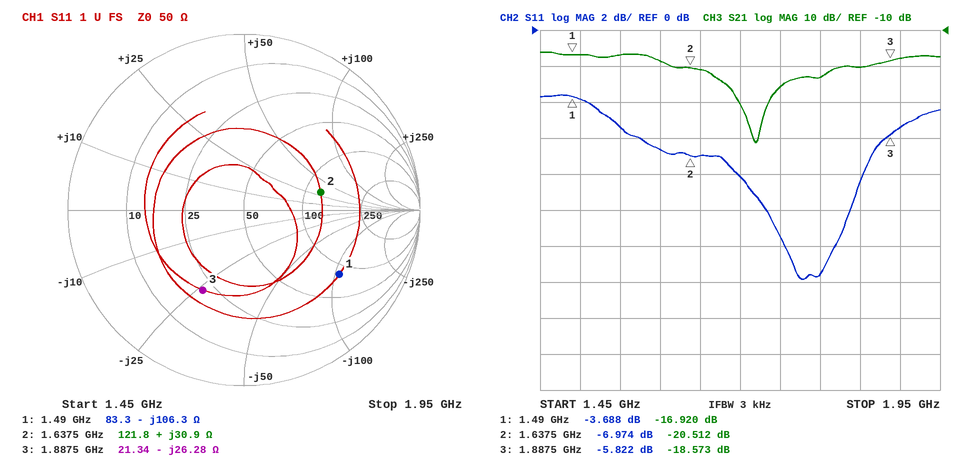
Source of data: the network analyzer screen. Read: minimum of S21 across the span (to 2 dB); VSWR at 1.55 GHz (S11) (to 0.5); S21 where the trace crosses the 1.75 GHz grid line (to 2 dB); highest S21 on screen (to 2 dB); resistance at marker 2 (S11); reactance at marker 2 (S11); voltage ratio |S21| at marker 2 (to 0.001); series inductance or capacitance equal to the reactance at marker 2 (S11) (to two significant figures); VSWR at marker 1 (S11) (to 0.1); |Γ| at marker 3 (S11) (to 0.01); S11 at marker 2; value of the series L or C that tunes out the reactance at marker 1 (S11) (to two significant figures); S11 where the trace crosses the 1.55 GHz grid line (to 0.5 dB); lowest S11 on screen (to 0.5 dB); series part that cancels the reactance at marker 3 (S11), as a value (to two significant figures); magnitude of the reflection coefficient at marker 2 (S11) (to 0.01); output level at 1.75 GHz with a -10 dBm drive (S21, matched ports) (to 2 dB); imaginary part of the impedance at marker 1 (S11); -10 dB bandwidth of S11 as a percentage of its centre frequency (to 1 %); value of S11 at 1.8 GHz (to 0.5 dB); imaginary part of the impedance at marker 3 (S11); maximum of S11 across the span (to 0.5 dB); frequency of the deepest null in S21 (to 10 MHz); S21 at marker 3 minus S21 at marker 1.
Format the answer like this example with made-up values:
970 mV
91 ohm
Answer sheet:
-42 dB
3.5
-26 dB
-16 dB
121.8 Ω
+30.9 Ω
0.094
3.0 nH
4.8
0.51
-6.974 dB
11 nH
-5.5 dB
-14.0 dB
2.2 nH
0.45
-36 dBm
-106.3 Ω
6 %
-13.5 dB
-26.28 Ω
-3.5 dB
1.72 GHz
-1.653 dB
